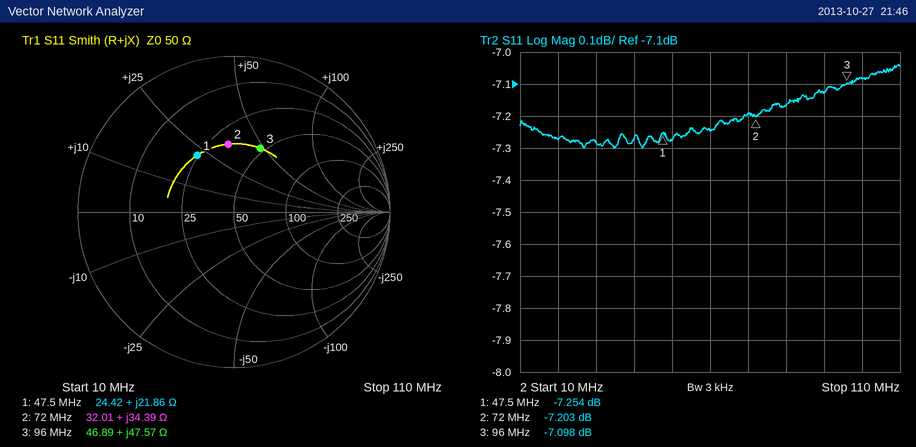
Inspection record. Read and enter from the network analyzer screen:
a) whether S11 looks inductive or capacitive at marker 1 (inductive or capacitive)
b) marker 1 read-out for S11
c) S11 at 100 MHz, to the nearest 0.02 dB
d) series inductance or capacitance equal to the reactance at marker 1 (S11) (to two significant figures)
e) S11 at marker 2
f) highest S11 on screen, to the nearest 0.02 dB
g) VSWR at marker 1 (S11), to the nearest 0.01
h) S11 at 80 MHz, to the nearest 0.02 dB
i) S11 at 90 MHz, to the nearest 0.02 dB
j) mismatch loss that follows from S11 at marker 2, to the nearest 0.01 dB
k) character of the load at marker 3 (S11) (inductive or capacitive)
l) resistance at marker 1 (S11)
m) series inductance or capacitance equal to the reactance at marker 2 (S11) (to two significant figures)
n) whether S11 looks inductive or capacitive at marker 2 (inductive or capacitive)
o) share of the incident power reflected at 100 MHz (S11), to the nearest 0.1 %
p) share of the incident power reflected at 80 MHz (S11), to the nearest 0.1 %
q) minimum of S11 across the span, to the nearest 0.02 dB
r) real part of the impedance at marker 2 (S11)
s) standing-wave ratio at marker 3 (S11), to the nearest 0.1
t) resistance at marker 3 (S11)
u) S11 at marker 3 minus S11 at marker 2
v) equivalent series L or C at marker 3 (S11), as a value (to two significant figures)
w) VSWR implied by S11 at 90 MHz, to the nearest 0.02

inductive
-7.254 dB
-7.08 dB
73 nH
-7.203 dB
-7.04 dB
2.53
-7.16 dB
-7.12 dB
0.92 dB
inductive
24.42 Ω
76 nH
inductive
19.6 %
19.2 %
-7.30 dB
32.01 Ω
2.6
46.89 Ω
0.105 dB
79 nH
2.58
